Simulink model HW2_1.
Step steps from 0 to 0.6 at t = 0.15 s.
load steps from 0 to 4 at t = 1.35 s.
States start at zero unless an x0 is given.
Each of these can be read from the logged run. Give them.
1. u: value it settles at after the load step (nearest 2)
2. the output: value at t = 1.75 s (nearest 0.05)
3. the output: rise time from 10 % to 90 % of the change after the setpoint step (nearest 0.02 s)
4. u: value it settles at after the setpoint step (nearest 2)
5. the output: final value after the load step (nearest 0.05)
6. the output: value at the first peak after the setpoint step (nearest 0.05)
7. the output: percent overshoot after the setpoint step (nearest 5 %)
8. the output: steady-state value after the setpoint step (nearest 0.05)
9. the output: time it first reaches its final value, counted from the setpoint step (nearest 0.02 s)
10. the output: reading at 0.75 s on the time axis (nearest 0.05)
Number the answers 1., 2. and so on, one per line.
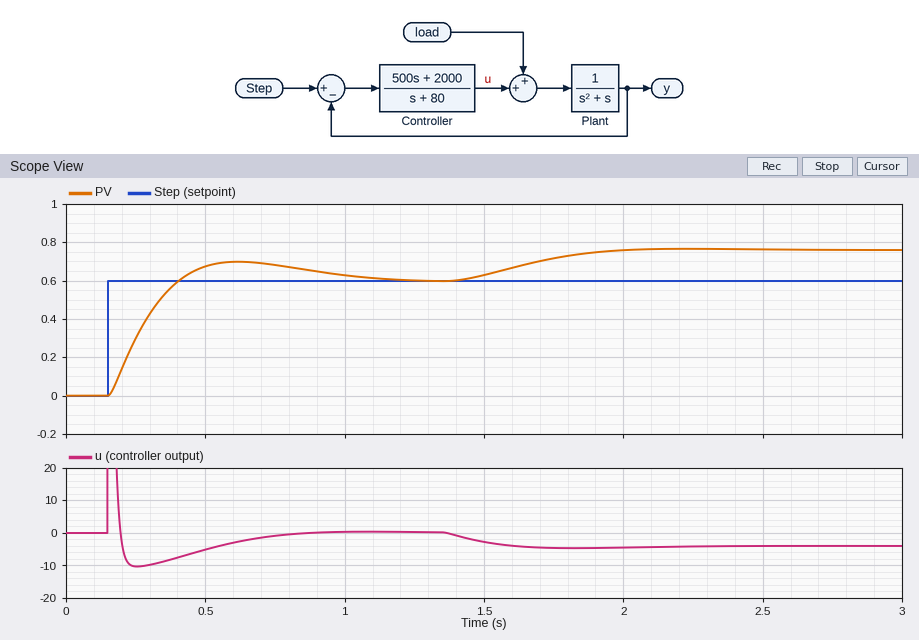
1. -4
2. 0.70
3. 0.18 s
4. 0
5. 0.75
6. 0.70
7. 15 %
8. 0.60
9. 0.26 s
10. 0.70
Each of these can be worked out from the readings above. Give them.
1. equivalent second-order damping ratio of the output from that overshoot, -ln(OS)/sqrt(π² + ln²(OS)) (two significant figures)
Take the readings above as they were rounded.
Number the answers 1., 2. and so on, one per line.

1. 0.52
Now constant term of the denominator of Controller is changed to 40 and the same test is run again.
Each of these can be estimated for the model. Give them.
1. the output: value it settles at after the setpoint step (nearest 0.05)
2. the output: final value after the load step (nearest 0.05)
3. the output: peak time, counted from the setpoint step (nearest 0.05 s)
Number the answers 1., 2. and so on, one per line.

1. 0.60
2. 0.70
3. 0.25 s
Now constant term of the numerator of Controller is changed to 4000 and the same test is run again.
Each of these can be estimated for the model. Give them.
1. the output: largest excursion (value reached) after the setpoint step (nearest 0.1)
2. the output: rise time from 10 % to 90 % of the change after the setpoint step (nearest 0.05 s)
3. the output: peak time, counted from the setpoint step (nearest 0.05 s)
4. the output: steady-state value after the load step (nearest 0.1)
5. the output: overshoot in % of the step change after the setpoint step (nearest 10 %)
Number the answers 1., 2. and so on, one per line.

1. 0.8
2. 0.15 s
3. 0.35 s
4. 0.7
5. 30 %
